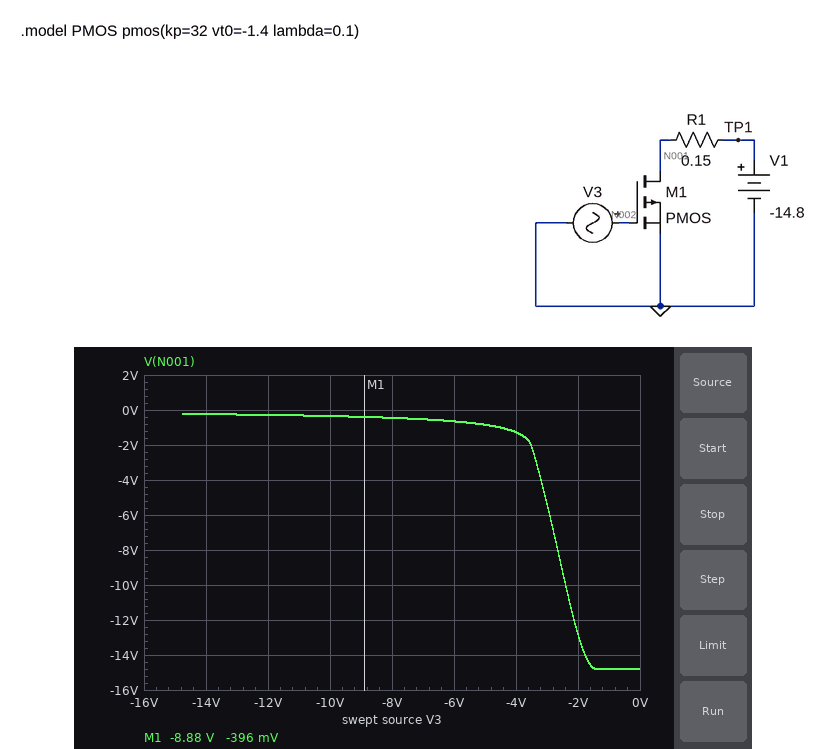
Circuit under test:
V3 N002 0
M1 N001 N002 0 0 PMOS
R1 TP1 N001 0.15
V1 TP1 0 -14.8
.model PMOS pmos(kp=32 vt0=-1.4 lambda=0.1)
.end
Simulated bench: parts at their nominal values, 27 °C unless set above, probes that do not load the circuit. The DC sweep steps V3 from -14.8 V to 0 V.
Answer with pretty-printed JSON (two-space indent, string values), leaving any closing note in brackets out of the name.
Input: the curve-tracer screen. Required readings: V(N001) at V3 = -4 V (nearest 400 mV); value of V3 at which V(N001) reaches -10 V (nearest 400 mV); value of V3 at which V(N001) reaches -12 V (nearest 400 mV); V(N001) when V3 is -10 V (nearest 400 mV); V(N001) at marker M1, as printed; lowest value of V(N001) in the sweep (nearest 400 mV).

{
  "V(N001) at V3 = -4 V": "-1.2 V",
  "value of V3 at which V(N001) reaches -10 V": "-2.4 V",
  "value of V3 at which V(N001) reaches -12 V": "-2.0 V",
  "V(N001) when V3 is -10 V": "-400 mV",
  "V(N001) at marker M1, as printed": "-396 mV",
  "lowest value of V(N001) in the sweep": "-14.8 V"
}
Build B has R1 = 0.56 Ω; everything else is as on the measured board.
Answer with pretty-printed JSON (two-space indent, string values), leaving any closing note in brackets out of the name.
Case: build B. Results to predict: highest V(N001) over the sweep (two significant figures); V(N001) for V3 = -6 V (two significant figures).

{
  "highest V(N001) over the sweep": "-61 mV",
  "V(N001) for V3 = -6 V": "-180 mV"
}
